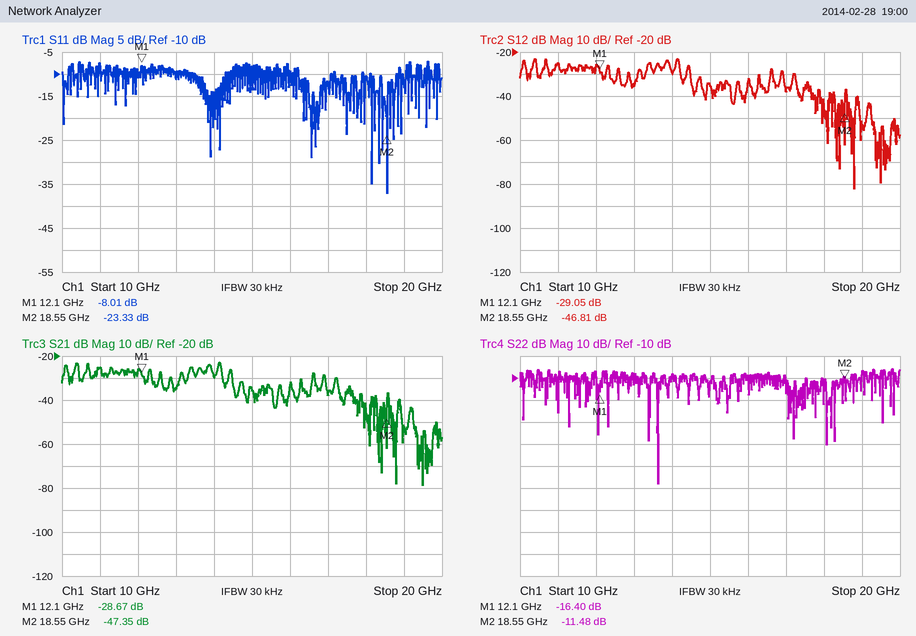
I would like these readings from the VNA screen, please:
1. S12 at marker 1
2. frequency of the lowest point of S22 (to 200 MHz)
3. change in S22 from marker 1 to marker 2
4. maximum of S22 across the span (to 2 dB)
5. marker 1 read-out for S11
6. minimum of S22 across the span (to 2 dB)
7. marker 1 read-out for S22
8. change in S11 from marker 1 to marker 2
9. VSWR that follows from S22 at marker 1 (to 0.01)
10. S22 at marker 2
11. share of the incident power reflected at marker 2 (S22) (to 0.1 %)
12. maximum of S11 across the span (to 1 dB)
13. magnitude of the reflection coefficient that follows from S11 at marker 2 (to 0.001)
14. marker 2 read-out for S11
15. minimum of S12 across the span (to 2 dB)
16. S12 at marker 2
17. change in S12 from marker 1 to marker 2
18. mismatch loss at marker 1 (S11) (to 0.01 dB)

-29.05 dB
13.6 GHz
4.92 dB
-6 dB
-8.01 dB
-58 dB
-16.40 dB
-15.32 dB
1.36
-11.48 dB
7.1 %
-7 dB
0.068
-23.33 dB
-82 dB
-46.81 dB
-17.76 dB
0.75 dB
